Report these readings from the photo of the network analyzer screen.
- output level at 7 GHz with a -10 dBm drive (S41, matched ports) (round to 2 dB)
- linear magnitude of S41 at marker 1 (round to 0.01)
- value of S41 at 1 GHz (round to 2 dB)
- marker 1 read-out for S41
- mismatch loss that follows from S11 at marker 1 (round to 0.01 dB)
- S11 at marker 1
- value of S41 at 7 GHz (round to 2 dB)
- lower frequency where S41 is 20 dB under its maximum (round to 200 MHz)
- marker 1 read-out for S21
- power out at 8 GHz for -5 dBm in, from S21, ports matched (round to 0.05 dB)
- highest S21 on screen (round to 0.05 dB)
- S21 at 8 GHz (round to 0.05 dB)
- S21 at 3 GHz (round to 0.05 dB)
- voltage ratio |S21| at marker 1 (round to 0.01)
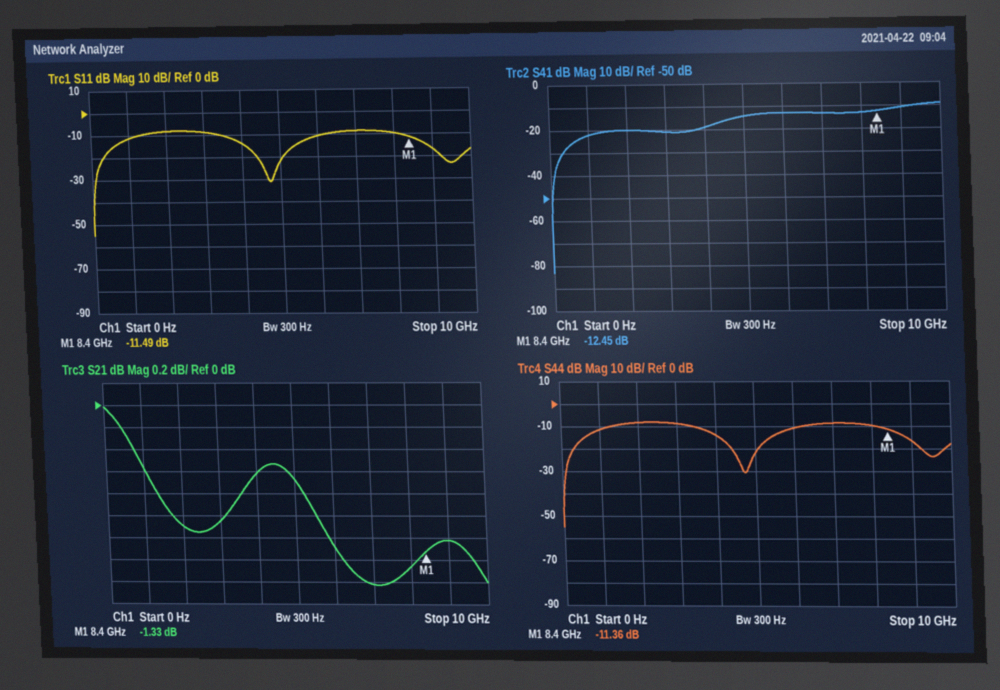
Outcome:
-24 dBm
0.24
-22 dB
-12.45 dB
0.32 dB
-11.49 dB
-14 dB
400 MHz
-1.33 dB
-6.45 dBm
0.00 dB
-1.45 dB
-1.05 dB
0.86
